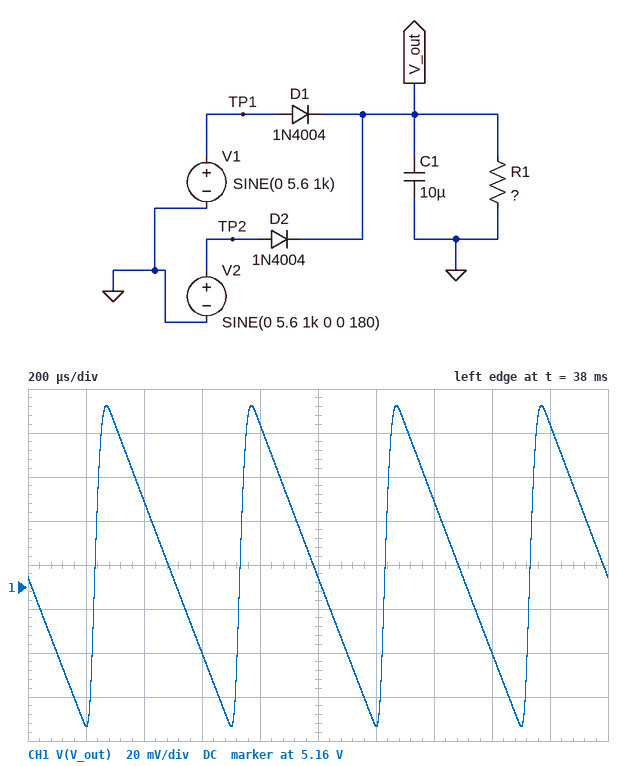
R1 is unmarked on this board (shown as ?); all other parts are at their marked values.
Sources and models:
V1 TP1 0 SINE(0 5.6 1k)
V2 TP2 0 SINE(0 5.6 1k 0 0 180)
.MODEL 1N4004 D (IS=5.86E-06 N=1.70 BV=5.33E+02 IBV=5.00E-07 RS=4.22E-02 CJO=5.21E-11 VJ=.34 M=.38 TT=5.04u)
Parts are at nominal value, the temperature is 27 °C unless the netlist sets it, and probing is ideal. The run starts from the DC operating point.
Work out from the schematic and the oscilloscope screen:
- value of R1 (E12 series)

1.5 kΩ
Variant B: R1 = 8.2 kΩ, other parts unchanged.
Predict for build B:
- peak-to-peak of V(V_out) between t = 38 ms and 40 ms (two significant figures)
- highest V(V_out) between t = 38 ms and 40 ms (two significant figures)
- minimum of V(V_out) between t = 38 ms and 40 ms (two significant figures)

28 mV
5.3 V
5.3 V
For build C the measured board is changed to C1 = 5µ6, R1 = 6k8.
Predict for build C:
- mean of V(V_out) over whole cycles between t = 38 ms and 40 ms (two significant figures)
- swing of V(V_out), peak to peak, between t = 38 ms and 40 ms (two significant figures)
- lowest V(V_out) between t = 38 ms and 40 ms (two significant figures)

5.3 V
60 mV
5.2 V
